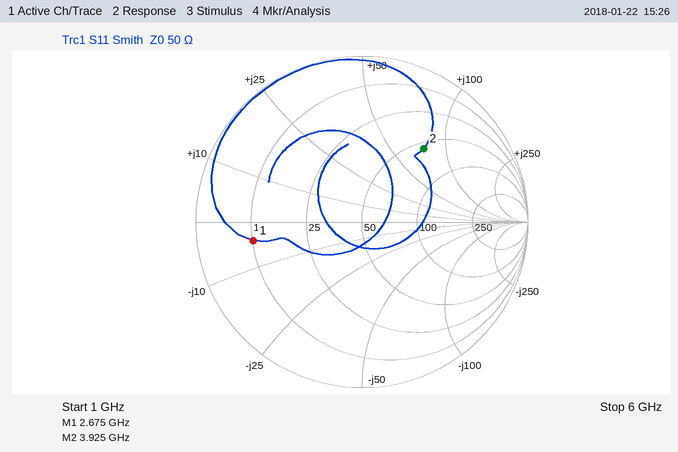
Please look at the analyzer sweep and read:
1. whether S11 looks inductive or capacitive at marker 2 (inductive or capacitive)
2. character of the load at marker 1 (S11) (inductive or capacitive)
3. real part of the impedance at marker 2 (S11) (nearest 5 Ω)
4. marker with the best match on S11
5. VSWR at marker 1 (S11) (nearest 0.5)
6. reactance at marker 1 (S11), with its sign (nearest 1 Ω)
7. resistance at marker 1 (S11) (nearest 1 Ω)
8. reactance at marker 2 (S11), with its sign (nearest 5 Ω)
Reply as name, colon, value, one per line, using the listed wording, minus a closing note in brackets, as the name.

whether S11 looks inductive or capacitive at marker 2: inductive
character of the load at marker 1 (S11): capacitive
real part of the impedance at marker 2 (S11): 55 Ω
marker with the best match on S11: marker 2
VSWR at marker 1 (S11): 5.0
reactance at marker 1 (S11), with its sign: -4 Ω
resistance at marker 1 (S11): 10 Ω
reactance at marker 2 (S11), with its sign: +75 Ω
